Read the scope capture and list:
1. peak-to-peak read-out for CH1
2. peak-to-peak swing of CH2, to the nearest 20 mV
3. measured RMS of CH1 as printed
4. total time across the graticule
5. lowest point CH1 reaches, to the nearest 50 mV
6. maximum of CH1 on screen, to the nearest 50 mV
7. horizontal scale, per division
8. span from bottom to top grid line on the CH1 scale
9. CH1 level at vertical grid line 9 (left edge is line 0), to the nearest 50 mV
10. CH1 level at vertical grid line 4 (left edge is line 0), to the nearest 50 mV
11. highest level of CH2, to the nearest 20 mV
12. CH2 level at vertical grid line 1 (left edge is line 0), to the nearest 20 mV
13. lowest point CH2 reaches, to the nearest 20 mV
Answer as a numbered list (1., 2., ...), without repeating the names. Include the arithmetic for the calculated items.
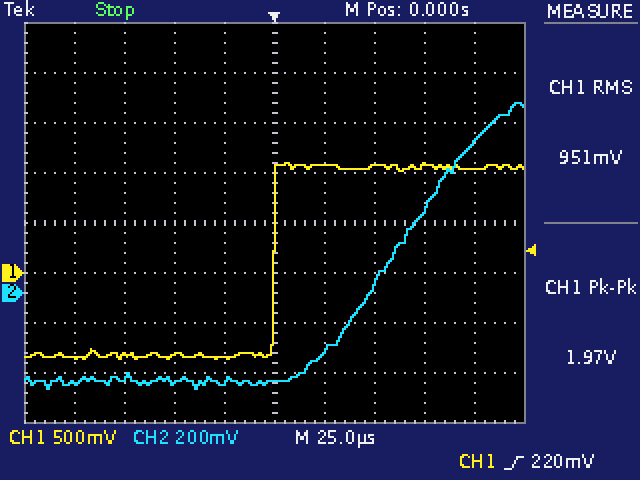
1. 1.97 V
2. 760 mV − (-380 mV) = 1.14 V
3. 951 mV
4. 250 µs
5. -850 mV
6. 1.10 V
7. 25 µs
8. 4 V
9. 1.05 V
10. -850 mV
11. 760 mV
12. -360 mV
13. -380 mV
